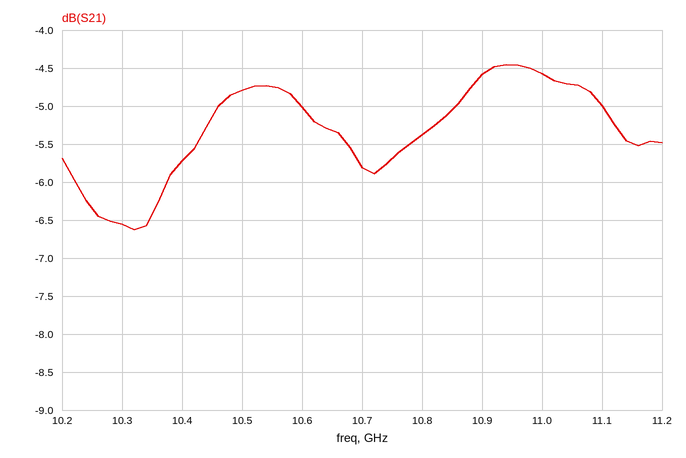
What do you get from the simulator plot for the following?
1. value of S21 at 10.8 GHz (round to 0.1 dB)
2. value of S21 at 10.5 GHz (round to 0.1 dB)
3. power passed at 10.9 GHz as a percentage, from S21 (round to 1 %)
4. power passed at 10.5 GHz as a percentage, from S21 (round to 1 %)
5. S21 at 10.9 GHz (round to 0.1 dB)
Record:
-5.4 dB
-4.8 dB
35 %
33 %
-4.6 dB
